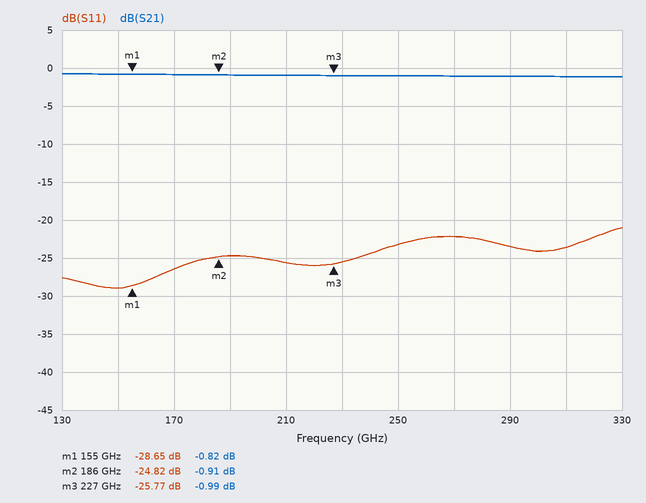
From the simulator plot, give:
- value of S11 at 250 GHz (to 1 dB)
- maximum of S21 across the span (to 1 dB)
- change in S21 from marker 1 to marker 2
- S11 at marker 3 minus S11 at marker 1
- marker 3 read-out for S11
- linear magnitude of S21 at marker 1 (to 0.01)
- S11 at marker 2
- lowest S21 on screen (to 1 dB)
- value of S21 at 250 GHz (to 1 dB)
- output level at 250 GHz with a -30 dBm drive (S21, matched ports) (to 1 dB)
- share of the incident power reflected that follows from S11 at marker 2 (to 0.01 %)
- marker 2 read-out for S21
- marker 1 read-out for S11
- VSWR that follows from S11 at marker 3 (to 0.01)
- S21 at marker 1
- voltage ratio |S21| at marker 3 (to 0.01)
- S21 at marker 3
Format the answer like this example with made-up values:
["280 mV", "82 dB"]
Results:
["-23 dB", "-1 dB", "-0.09 dB", "2.88 dB", "-25.77 dB", "0.91", "-24.82 dB", "-1 dB", "-1 dB", "-31 dBm", "0.33 %", "-0.91 dB", "-28.65 dB", "1.11", "-0.82 dB", "0.89", "-0.99 dB"]
